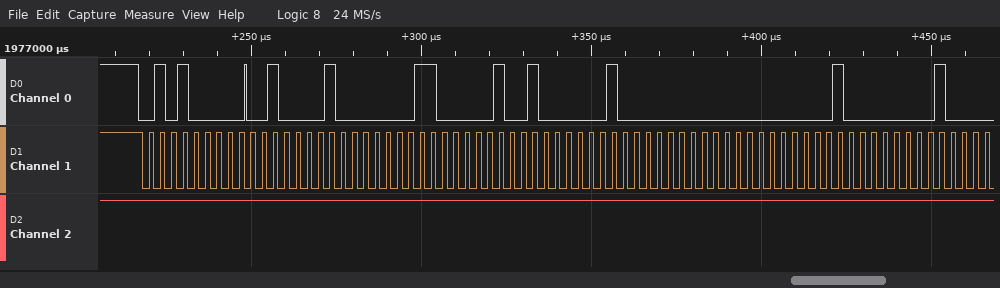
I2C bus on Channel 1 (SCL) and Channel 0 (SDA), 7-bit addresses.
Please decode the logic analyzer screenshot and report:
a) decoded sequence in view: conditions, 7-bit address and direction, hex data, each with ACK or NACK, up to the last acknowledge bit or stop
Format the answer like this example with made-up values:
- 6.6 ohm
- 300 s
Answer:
- start, address 28 write ACK, 21 ACK, 03 ACK, 09 ACK, 04 ACK, 00 ACK, 01 ACK, 01 ACK
